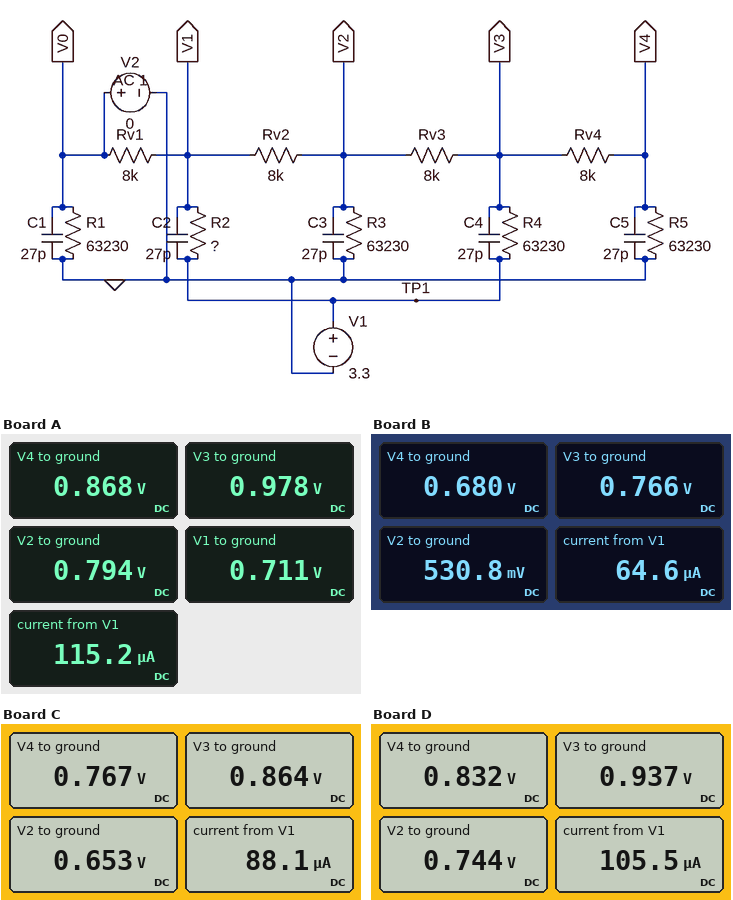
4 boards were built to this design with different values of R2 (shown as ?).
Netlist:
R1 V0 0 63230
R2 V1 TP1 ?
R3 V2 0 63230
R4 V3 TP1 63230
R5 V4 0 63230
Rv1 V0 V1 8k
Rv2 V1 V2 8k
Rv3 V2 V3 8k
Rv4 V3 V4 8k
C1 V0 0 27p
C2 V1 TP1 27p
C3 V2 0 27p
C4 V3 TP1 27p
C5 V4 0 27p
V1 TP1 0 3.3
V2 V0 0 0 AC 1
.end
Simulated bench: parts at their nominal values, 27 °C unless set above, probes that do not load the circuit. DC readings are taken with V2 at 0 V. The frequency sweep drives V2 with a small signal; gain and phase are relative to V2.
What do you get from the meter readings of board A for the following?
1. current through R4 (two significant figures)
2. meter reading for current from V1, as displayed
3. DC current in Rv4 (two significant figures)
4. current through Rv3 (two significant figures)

37 µA
115.2 µA
14 µA
23 µA
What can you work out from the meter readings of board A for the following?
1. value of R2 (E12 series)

33 kΩ
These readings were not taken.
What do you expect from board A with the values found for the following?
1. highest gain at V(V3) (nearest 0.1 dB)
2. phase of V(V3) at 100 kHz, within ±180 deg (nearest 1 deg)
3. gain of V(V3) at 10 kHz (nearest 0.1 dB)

-7.7 dB
-33 deg
-7.7 dB
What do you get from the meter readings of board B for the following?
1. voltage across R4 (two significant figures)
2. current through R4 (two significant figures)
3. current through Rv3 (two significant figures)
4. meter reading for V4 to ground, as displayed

2.5 V
40 µA
29 µA
0.680 V
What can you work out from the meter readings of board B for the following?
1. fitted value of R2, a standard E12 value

120 kΩ
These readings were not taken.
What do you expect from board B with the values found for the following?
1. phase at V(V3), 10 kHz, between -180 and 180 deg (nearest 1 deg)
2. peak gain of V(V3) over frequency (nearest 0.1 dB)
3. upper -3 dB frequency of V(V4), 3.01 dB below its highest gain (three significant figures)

-4 deg
-6.6 dB
170 kHz
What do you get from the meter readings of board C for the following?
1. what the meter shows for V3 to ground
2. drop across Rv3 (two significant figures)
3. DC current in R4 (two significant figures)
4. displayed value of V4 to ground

0.864 V
210 mV
39 µA
0.767 V
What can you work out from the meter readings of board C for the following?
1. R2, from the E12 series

56 kΩ
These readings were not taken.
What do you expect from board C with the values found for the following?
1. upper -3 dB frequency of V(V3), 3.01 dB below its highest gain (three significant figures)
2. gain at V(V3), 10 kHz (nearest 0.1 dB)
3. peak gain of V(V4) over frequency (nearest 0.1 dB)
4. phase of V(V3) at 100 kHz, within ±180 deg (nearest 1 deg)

180 kHz
-7.1 dB
-8.1 dB
-34 deg
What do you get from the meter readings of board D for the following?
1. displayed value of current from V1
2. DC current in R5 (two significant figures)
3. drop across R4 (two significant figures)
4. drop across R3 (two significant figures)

105.5 µA
13 µA
2.4 V
740 mV
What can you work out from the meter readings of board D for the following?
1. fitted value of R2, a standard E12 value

39 kΩ
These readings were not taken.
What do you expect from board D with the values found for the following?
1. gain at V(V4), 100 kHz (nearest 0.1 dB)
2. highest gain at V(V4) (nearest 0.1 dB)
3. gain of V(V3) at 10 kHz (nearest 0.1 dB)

-9.7 dB
-8.5 dB
-7.5 dB
